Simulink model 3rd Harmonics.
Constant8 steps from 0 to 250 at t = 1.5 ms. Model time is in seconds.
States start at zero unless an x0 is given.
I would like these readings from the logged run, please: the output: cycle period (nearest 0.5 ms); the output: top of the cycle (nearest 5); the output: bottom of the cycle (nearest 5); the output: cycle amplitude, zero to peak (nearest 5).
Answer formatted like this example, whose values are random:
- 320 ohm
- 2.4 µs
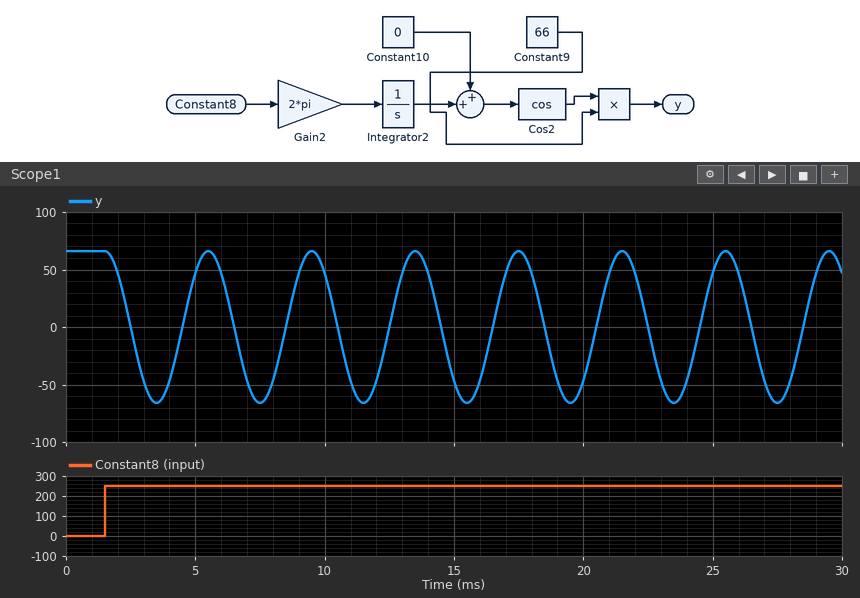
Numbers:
- 4.0 ms
- 65
- -65
- 65
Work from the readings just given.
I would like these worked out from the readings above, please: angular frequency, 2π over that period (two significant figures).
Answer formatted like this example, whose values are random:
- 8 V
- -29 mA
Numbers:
- 1.6 rad/ms
